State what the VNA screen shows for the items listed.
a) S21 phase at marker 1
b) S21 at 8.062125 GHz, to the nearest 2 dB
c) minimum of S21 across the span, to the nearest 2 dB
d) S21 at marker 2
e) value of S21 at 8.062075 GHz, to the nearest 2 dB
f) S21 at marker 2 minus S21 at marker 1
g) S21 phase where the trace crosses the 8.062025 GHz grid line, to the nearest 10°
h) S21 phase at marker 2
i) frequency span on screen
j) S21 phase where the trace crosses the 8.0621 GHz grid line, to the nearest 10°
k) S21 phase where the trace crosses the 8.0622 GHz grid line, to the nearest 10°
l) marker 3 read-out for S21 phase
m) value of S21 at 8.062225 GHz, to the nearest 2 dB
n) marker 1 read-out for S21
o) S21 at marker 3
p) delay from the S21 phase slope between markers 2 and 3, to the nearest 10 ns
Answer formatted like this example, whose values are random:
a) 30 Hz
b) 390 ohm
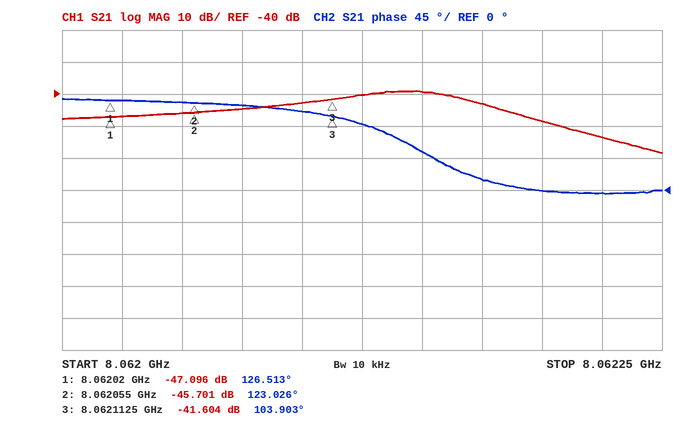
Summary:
a) 126.513°
b) -40 dB
c) -58 dB
d) -45.701 dB
e) -44 dB
f) 1.395 dB
g) 130°
h) 123.026°
i) 250 kHz
j) 110°
k) 0°
l) 103.903°
m) -54 dB
n) -47.096 dB
o) -41.604 dB
p) 920 ns
